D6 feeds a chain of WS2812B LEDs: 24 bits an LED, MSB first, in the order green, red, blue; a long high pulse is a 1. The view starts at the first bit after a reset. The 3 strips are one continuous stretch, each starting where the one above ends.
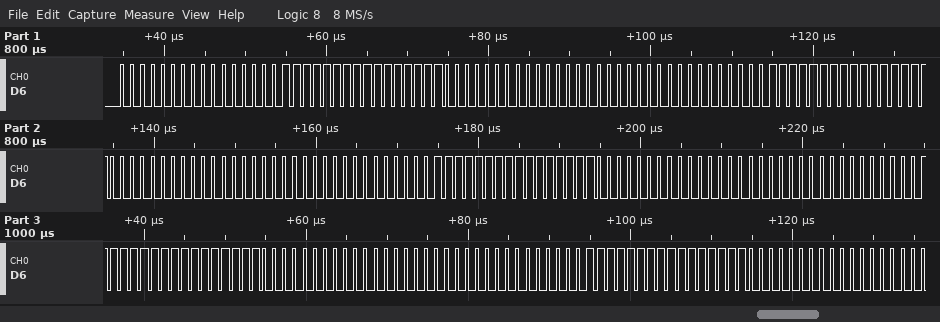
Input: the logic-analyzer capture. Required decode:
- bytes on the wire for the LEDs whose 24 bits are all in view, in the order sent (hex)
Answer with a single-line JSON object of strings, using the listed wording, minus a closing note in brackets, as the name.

{"bytes on the wire for the LEDs whose 24 bits are all in view, in the order sent": "00 00 FF FF 00 00 00 00 FF FF 00 00 00 00 FF FF 00 00 00 00 FF FF 00 00 00 00 FF FF 00 00"}
